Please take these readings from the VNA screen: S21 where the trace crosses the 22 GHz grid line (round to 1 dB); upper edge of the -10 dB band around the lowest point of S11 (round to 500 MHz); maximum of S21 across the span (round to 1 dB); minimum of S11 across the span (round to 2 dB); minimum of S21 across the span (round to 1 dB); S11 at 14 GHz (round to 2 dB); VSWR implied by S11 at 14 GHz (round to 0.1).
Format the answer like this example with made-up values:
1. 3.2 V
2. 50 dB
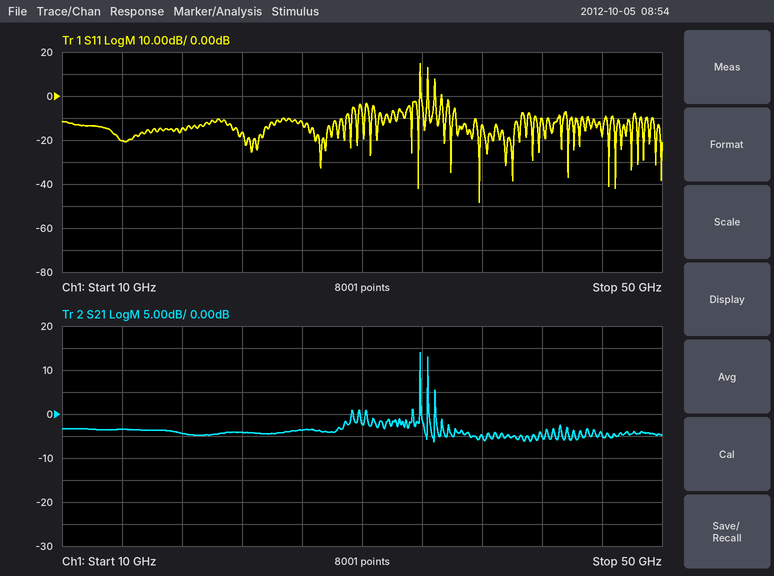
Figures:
1. -4 dB
2. 40.5 GHz
3. 14 dB
4. -48 dB
5. -6 dB
6. -20 dB
7. 1.2
